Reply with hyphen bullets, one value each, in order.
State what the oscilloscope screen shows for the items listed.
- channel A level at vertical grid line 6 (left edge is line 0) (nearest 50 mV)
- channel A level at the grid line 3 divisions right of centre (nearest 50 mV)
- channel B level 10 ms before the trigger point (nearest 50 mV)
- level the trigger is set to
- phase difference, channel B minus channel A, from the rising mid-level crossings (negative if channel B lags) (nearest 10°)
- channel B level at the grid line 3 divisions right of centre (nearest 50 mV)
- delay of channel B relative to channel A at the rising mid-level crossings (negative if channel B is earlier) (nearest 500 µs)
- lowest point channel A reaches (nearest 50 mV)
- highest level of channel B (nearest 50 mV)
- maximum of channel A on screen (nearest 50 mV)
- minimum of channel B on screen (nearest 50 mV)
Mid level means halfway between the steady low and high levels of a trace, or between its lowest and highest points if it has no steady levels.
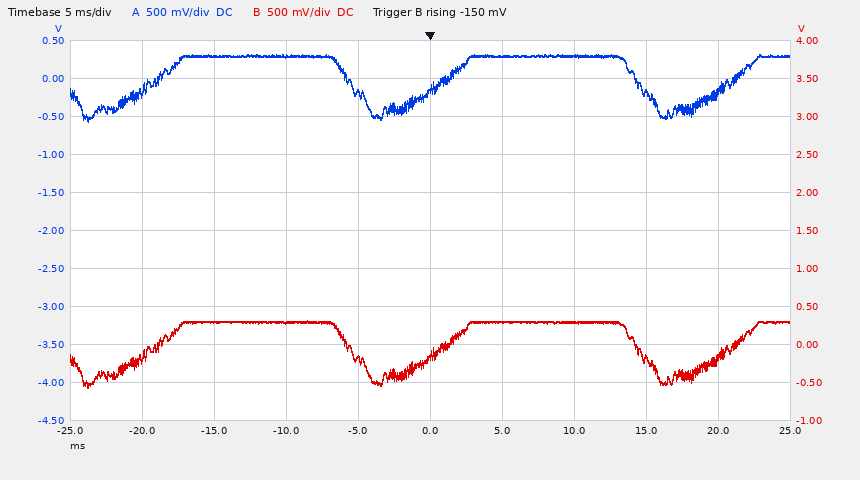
- 300 mV
- -200 mV
- 300 mV
- -150 mV
- 0°
- -200 mV
- 0.0 ms
- -550 mV
- 300 mV
- 300 mV
- -550 mV
